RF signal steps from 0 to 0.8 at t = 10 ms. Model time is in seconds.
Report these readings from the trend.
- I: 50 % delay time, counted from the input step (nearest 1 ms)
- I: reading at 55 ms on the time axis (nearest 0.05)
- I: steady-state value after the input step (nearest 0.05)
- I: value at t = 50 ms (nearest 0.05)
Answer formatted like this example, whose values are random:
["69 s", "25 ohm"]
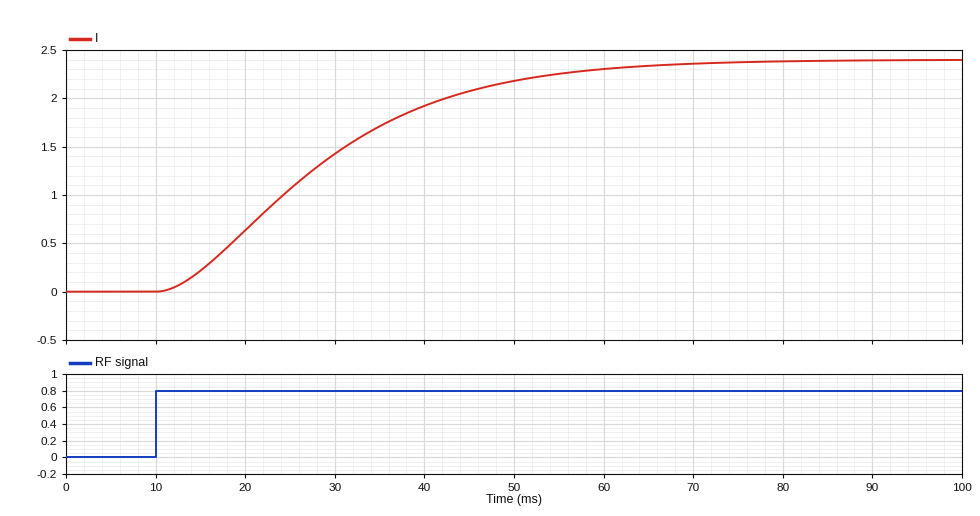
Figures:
["17 ms", "2.25", "2.40", "2.20"]
